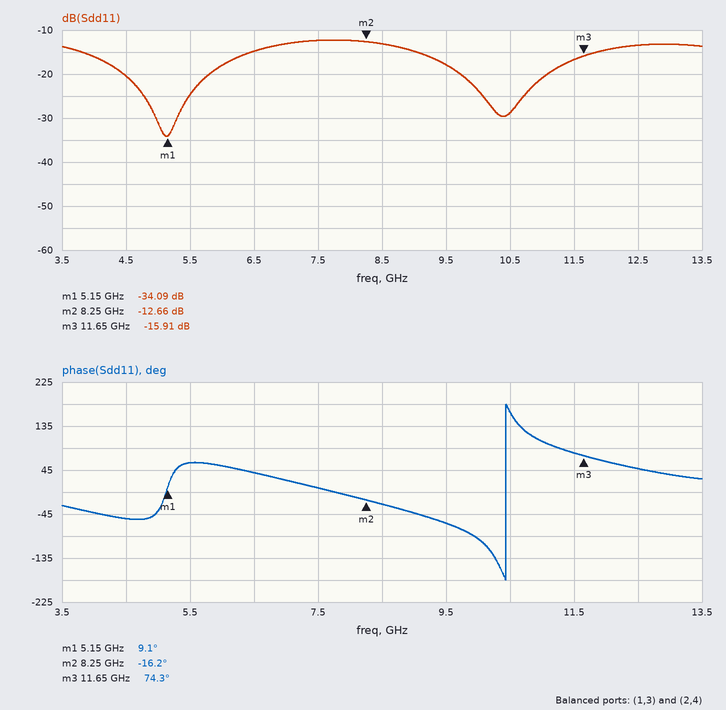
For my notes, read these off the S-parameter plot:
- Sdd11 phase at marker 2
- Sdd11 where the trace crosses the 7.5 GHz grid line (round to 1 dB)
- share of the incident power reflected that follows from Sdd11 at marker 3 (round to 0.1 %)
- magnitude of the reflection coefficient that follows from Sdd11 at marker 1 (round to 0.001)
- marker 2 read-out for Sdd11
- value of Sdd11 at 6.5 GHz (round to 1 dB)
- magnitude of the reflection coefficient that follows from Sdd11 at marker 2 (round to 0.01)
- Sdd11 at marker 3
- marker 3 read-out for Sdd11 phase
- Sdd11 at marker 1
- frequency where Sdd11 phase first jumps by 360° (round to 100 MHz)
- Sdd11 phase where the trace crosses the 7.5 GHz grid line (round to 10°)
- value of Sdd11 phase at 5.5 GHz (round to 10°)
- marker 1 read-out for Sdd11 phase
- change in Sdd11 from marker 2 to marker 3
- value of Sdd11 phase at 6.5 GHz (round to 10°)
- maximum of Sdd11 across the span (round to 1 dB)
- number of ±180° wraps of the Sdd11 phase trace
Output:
-16.2°
-12 dB
2.6 %
0.020
-12.66 dB
-15 dB
0.23
-15.91 dB
74.3°
-34.09 dB
10.4 GHz
10°
60°
9.1°
-3.25 dB
40°
-12 dB
1
